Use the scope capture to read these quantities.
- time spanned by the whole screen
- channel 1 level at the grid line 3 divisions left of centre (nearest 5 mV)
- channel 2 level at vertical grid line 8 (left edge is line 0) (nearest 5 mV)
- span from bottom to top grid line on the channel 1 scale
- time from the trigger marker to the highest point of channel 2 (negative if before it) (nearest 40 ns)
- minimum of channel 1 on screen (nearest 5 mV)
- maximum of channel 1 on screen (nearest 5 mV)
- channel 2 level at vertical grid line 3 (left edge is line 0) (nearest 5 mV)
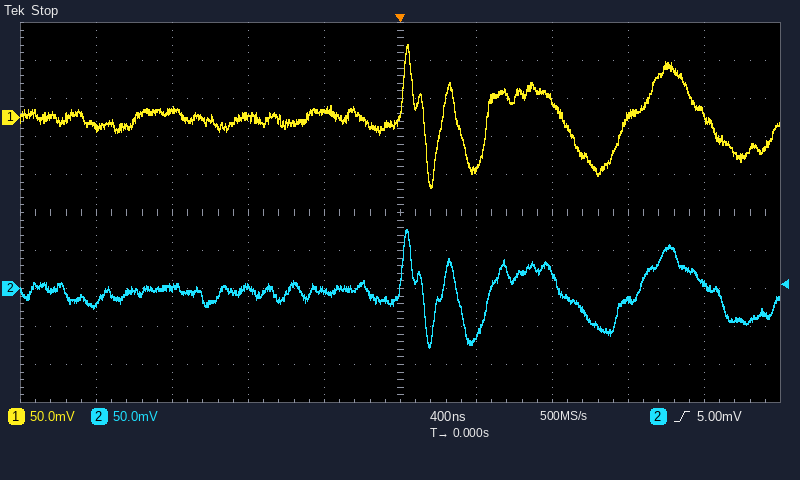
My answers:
4 µs
10 mV
-15 mV
500 mV
+40 ns
-90 mV
95 mV
0 mV
